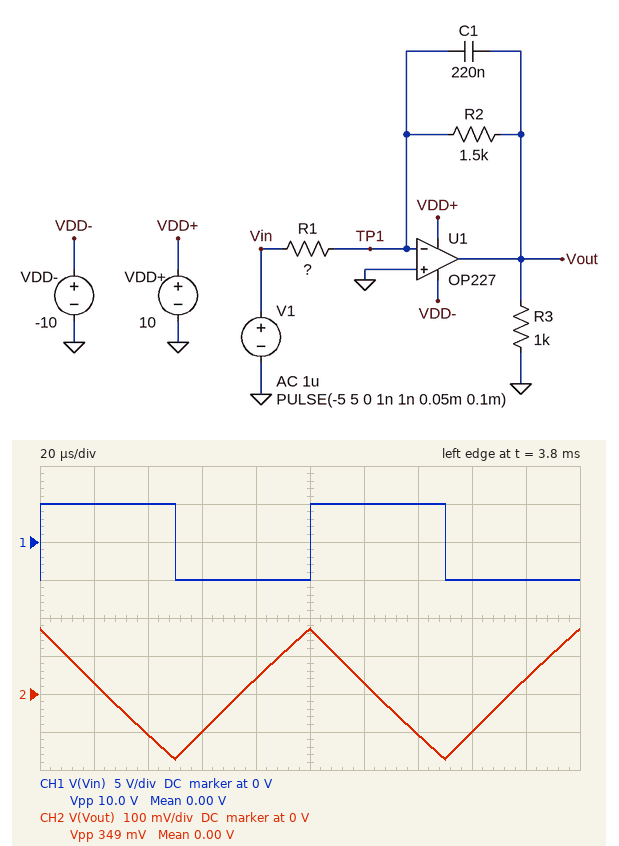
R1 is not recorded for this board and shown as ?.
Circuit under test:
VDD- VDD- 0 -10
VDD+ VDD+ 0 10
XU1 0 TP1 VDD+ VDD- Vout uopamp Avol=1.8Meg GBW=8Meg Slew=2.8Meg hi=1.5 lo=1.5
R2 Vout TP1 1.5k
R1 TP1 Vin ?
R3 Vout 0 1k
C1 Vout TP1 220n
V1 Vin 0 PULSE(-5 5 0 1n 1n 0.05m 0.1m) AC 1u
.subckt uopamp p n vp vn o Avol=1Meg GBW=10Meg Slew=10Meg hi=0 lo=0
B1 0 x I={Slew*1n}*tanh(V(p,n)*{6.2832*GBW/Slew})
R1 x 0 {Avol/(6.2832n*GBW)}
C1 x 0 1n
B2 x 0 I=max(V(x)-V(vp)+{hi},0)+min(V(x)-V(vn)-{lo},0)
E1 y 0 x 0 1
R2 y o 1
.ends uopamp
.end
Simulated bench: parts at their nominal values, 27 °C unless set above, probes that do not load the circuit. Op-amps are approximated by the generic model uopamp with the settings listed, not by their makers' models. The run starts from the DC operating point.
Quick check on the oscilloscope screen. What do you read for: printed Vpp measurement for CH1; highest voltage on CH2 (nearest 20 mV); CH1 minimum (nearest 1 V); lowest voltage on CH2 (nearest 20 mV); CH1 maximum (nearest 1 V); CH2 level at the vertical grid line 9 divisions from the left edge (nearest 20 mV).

10.0 V
180 mV
-5 V
-180 mV
5 V
40 mV
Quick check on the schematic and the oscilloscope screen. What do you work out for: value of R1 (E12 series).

3.3 kΩ
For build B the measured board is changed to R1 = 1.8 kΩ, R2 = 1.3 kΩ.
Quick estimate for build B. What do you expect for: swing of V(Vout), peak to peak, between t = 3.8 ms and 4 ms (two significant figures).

640 mV
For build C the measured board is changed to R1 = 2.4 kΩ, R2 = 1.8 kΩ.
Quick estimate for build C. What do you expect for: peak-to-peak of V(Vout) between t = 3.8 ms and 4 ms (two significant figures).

480 mV
